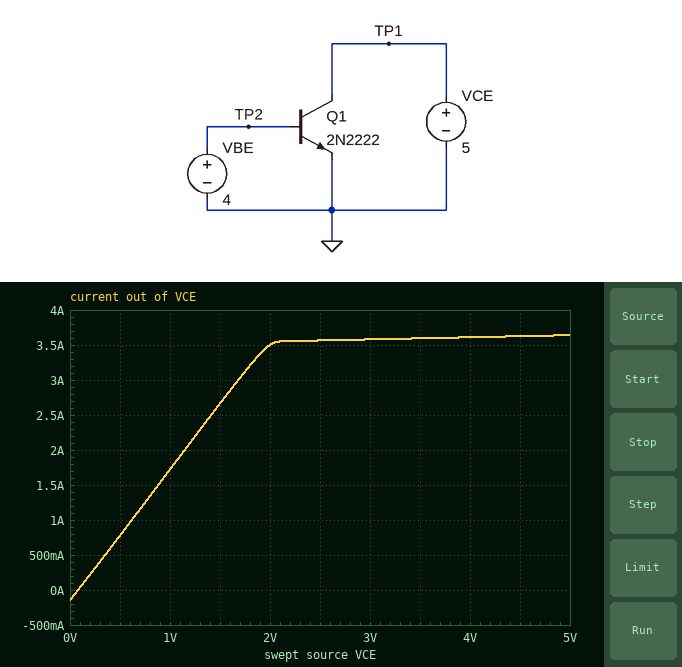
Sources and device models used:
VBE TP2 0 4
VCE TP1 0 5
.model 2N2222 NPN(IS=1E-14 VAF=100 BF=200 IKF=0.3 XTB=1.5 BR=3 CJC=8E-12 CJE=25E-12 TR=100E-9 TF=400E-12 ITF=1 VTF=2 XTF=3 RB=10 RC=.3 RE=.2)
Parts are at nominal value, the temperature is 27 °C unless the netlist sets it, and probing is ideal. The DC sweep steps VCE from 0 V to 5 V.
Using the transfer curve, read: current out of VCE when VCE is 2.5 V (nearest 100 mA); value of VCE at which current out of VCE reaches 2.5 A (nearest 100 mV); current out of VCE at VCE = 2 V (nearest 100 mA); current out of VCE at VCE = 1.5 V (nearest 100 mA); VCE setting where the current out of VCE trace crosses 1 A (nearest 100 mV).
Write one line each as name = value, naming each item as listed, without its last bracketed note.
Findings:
current out of VCE when VCE is 2.5 V = 3.6 A
value of VCE at which current out of VCE reaches 2.5 A = 1.4 V
current out of VCE at VCE = 2 V = 3.5 A
current out of VCE at VCE = 1.5 V = 2.7 A
VCE setting where the current out of VCE trace crosses 1 A = 600 mV
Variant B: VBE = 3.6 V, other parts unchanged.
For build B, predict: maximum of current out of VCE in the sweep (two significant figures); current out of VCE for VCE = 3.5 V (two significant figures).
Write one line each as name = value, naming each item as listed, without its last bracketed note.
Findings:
maximum of current out of VCE in the sweep = 3.4 A
current out of VCE for VCE = 3.5 V = 3.3 A
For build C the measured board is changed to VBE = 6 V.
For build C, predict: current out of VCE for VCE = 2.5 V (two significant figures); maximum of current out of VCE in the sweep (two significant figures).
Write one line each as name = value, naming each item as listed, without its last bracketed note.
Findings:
current out of VCE for VCE = 2.5 V = 4.5 A
maximum of current out of VCE in the sweep = 4.8 A
